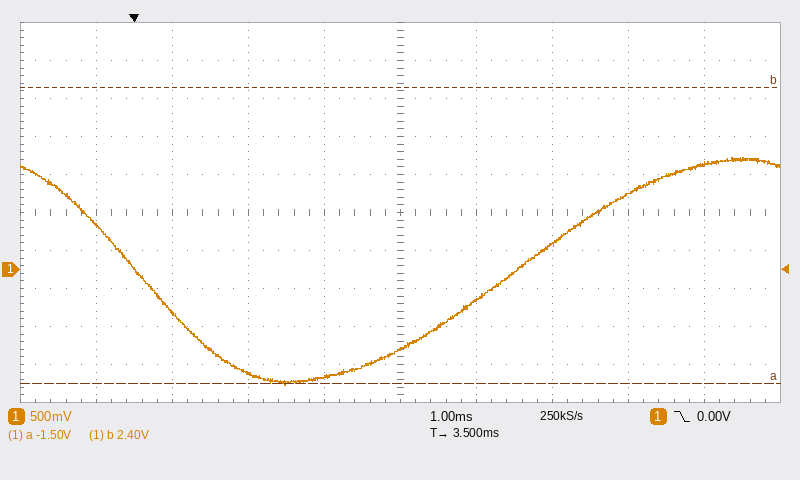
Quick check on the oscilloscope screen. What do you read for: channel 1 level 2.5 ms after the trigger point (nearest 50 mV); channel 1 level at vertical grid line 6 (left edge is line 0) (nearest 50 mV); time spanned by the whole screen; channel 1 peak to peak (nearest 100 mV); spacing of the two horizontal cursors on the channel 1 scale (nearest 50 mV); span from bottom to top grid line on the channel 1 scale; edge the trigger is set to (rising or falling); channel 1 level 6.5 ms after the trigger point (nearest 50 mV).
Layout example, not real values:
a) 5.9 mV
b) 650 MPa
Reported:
a) -1.40 V
b) -400 mV
c) 10 ms
d) 3.00 V
e) 3.90 V
f) 5 V
g) falling
h) 1.00 V
